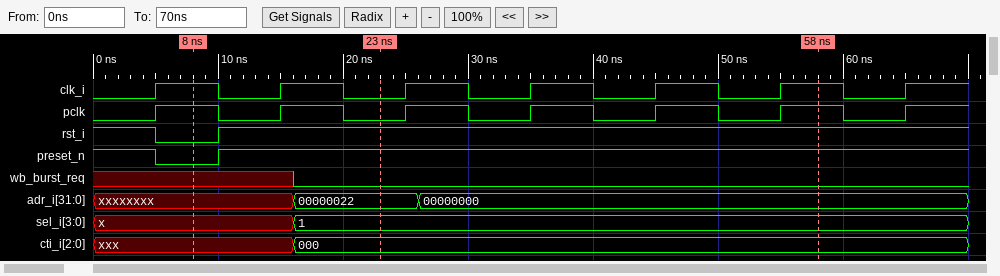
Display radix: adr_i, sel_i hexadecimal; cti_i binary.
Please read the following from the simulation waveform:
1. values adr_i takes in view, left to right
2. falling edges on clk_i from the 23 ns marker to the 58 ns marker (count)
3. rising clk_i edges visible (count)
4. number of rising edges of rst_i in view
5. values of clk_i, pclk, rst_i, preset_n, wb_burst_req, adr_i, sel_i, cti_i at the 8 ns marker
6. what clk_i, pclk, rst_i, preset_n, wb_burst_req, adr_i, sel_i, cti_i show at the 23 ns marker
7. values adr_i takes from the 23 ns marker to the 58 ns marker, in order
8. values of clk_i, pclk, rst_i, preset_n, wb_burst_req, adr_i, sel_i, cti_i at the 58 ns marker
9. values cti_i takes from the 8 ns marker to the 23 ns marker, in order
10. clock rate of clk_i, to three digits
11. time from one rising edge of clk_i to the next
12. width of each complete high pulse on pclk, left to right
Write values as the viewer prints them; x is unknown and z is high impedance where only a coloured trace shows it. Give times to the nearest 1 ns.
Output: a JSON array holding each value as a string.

["xxxxxxxx, 00000022, 00000000", "3", "7", "1", "clk_i=1, pclk=1, rst_i=0, preset_n=0, wb_burst_req=x, adr_i=xxxxxxxx, sel_i=x, cti_i=xxx", "clk_i=0, pclk=0, rst_i=1, preset_n=1, wb_burst_req=0, adr_i=00000022, sel_i=1, cti_i=000", "00000022, 00000000", "clk_i=1, pclk=1, rst_i=1, preset_n=1, wb_burst_req=0, adr_i=00000000, sel_i=1, cti_i=000", "xxx, 000", "100 MHz", "10 ns", "5 ns, 5 ns, 5 ns, 5 ns, 5 ns, 5 ns"]
